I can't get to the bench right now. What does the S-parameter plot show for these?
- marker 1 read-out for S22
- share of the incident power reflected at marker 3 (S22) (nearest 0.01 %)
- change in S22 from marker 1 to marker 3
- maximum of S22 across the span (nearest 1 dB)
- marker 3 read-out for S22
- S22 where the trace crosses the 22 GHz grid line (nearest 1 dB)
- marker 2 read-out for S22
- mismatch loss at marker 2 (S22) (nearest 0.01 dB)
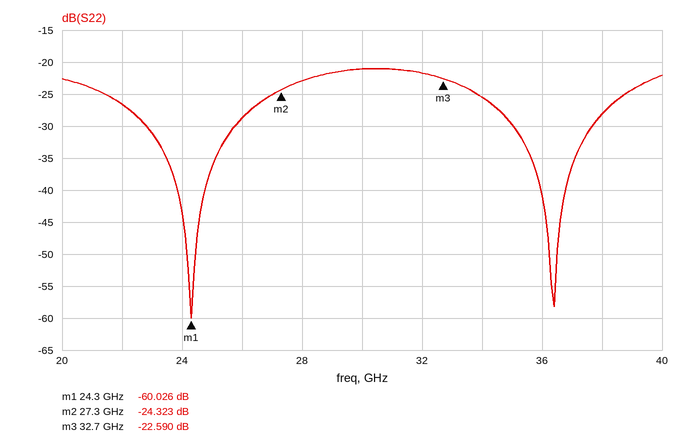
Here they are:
-60.026 dB
0.55 %
37.436 dB
-21 dB
-22.590 dB
-27 dB
-24.323 dB
0.02 dB
